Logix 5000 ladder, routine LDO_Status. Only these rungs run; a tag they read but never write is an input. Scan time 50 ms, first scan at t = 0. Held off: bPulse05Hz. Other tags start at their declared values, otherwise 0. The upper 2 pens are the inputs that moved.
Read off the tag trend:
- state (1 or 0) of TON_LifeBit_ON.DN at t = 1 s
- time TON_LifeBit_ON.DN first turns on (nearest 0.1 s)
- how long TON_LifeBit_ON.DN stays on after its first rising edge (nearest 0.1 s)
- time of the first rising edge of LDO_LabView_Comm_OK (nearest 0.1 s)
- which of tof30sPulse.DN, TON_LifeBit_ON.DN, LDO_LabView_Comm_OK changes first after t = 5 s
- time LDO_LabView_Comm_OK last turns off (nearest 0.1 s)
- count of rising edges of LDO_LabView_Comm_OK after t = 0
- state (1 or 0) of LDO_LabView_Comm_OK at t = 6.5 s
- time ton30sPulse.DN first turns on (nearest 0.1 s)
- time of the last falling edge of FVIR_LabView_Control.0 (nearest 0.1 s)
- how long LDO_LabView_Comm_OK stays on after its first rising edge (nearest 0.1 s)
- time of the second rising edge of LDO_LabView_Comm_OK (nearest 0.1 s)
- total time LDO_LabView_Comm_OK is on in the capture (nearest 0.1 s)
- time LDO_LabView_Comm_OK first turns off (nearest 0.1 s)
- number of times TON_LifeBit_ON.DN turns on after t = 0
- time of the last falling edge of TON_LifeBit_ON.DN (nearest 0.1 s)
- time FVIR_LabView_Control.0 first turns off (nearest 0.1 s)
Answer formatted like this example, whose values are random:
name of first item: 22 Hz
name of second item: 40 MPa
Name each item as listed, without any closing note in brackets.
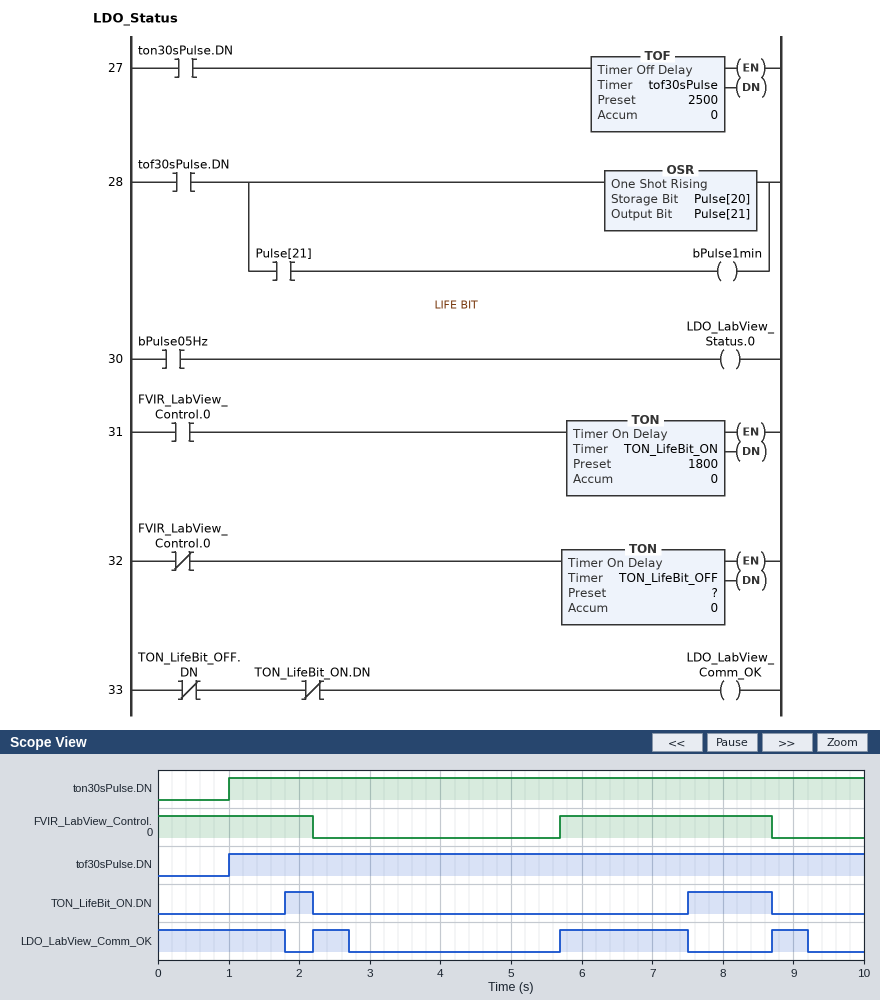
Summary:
state (1 or 0) of TON_LifeBit_ON.DN at t = 1 s: 0
time TON_LifeBit_ON.DN first turns on: 1.8 s
how long TON_LifeBit_ON.DN stays on after its first rising edge: 0.4 s
time of the first rising edge of LDO_LabView_Comm_OK: 2.2 s
which of tof30sPulse.DN, TON_LifeBit_ON.DN, LDO_LabView_Comm_OK changes first after t = 5 s: LDO_LabView_Comm_OK
time LDO_LabView_Comm_OK last turns off: 9.2 s
count of rising edges of LDO_LabView_Comm_OK after t = 0: 3
state (1 or 0) of LDO_LabView_Comm_OK at t = 6.5 s: 1
time ton30sPulse.DN first turns on: 1.0 s
time of the last falling edge of FVIR_LabView_Control.0: 8.7 s
how long LDO_LabView_Comm_OK stays on after its first rising edge: 0.5 s
time of the second rising edge of LDO_LabView_Comm_OK: 5.7 s
total time LDO_LabView_Comm_OK is on in the capture: 4.6 s
time LDO_LabView_Comm_OK first turns off: 1.8 s
number of times TON_LifeBit_ON.DN turns on after t = 0: 2
time of the last falling edge of TON_LifeBit_ON.DN: 8.7 s
time FVIR_LabView_Control.0 first turns off: 2.2 s
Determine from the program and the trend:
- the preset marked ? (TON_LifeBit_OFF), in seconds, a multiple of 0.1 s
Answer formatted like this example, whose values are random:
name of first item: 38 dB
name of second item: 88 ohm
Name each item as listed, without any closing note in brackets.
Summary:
the preset marked ? (TON_LifeBit_OFF), in seconds, a multiple of 0.1 s: 0.5 s
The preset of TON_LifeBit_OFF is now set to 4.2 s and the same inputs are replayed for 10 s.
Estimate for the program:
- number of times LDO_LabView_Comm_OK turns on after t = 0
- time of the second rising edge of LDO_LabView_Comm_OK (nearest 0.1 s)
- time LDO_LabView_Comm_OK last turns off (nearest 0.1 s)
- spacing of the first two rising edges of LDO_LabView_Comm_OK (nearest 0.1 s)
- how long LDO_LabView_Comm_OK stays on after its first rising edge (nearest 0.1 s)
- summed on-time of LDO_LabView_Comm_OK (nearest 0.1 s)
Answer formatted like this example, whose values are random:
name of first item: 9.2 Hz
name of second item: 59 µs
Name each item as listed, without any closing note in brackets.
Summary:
number of times LDO_LabView_Comm_OK turns on after t = 0: 2
time of the second rising edge of LDO_LabView_Comm_OK: 8.7 s
time LDO_LabView_Comm_OK last turns off: 7.5 s
spacing of the first two rising edges of LDO_LabView_Comm_OK: 6.5 s
how long LDO_LabView_Comm_OK stays on after its first rising edge: 5.3 s
summed on-time of LDO_LabView_Comm_OK: 8.4 s
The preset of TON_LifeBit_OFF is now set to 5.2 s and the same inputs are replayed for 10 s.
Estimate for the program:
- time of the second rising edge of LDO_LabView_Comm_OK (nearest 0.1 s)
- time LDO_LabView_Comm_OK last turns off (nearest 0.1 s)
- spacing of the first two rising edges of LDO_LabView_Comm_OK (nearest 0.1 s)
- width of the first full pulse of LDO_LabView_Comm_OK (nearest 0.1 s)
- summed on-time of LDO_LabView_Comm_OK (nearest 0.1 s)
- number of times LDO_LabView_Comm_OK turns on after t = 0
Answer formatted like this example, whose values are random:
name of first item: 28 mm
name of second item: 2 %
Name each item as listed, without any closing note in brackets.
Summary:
time of the second rising edge of LDO_LabView_Comm_OK: 8.7 s
time LDO_LabView_Comm_OK last turns off: 7.5 s
spacing of the first two rising edges of LDO_LabView_Comm_OK: 6.5 s
width of the first full pulse of LDO_LabView_Comm_OK: 5.3 s
summed on-time of LDO_LabView_Comm_OK: 8.4 s
number of times LDO_LabView_Comm_OK turns on after t = 0: 2
